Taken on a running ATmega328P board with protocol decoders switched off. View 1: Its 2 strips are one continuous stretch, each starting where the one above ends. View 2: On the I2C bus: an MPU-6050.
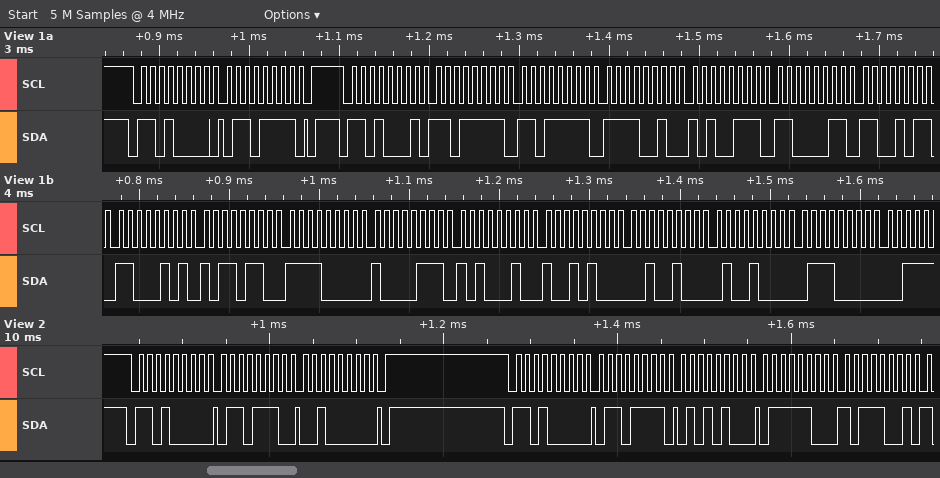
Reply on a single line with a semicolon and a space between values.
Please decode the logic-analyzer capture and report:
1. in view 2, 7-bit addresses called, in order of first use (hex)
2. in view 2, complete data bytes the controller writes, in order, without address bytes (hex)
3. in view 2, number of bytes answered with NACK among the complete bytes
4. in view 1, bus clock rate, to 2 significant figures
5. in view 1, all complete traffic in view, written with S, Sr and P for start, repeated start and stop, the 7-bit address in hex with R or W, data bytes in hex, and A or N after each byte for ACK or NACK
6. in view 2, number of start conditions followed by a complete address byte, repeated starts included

0x68; 6E 20 6F 54 7C B9; 0; 100 kHz; S 68W A 6F A P S 68R A DF A DF A F2 A A7 A C3 A CB A C5 A B6 A F0 A 87 A A2 A 94 A 24 A 48 A 70 A; 2
